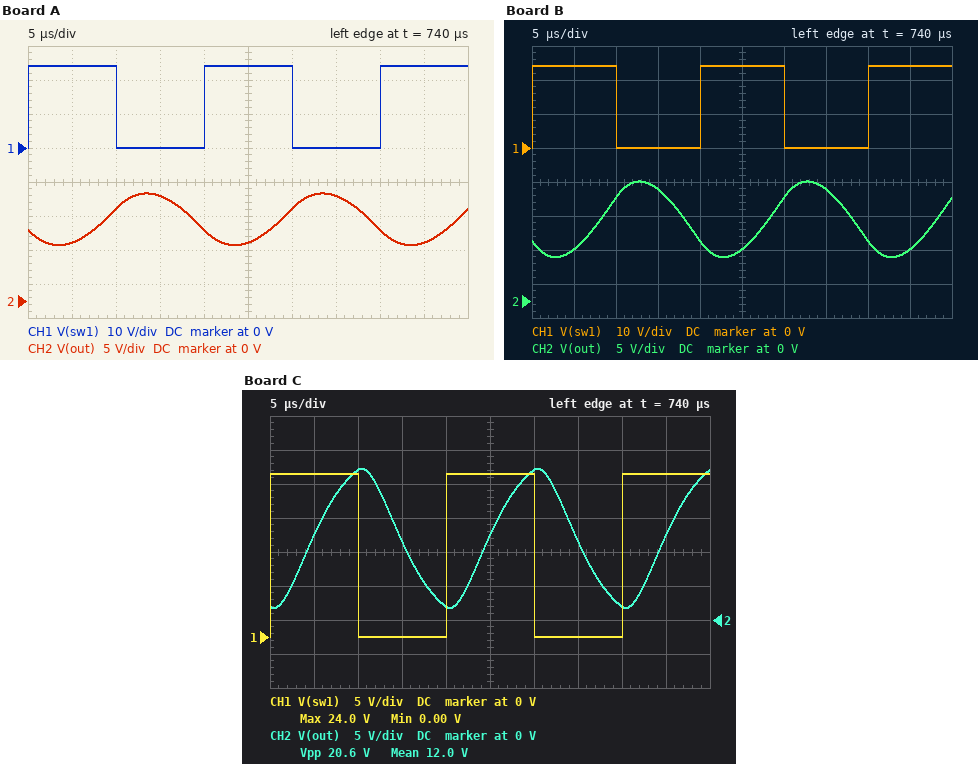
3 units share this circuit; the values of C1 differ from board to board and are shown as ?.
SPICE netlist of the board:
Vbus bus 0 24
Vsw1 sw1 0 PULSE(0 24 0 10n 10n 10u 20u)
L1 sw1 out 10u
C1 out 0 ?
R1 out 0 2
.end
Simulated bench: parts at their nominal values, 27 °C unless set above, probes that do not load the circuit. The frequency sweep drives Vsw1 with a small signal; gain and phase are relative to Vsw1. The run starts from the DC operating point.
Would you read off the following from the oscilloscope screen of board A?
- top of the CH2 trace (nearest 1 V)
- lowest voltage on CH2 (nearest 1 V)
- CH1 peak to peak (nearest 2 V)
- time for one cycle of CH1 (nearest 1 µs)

16 V
8 V
24 V
20 µs
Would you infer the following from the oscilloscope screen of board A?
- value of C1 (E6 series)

4.7 µF
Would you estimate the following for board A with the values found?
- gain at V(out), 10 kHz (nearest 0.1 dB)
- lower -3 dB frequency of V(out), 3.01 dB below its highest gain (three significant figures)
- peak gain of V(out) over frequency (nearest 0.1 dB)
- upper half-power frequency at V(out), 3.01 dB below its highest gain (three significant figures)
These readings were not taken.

1.2 dB
5.44 kHz
3.4 dB
27.6 kHz
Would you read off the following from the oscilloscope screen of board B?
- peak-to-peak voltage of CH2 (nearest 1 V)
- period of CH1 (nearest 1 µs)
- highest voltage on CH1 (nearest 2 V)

11 V
20 µs
24 V
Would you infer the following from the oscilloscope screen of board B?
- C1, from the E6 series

3.3 µF
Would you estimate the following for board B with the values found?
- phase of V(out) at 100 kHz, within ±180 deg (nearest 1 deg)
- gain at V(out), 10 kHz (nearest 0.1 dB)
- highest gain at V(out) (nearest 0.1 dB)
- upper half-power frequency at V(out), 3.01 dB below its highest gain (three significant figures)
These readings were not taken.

-165 deg
0.7 dB
2.1 dB
32.8 kHz
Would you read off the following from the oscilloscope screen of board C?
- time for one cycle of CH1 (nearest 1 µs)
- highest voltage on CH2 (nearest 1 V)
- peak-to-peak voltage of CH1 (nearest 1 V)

20 µs
22 V
24 V
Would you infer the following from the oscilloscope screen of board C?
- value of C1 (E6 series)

1 µF
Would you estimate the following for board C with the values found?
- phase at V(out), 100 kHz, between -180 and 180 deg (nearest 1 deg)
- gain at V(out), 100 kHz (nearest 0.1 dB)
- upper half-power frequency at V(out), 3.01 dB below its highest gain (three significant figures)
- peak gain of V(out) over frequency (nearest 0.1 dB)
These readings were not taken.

-133 deg
-12.7 dB
44.5 kHz
0 dB
